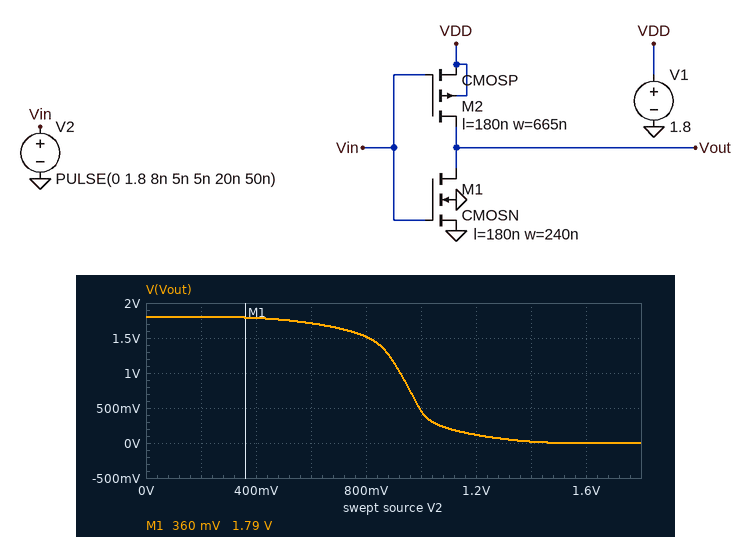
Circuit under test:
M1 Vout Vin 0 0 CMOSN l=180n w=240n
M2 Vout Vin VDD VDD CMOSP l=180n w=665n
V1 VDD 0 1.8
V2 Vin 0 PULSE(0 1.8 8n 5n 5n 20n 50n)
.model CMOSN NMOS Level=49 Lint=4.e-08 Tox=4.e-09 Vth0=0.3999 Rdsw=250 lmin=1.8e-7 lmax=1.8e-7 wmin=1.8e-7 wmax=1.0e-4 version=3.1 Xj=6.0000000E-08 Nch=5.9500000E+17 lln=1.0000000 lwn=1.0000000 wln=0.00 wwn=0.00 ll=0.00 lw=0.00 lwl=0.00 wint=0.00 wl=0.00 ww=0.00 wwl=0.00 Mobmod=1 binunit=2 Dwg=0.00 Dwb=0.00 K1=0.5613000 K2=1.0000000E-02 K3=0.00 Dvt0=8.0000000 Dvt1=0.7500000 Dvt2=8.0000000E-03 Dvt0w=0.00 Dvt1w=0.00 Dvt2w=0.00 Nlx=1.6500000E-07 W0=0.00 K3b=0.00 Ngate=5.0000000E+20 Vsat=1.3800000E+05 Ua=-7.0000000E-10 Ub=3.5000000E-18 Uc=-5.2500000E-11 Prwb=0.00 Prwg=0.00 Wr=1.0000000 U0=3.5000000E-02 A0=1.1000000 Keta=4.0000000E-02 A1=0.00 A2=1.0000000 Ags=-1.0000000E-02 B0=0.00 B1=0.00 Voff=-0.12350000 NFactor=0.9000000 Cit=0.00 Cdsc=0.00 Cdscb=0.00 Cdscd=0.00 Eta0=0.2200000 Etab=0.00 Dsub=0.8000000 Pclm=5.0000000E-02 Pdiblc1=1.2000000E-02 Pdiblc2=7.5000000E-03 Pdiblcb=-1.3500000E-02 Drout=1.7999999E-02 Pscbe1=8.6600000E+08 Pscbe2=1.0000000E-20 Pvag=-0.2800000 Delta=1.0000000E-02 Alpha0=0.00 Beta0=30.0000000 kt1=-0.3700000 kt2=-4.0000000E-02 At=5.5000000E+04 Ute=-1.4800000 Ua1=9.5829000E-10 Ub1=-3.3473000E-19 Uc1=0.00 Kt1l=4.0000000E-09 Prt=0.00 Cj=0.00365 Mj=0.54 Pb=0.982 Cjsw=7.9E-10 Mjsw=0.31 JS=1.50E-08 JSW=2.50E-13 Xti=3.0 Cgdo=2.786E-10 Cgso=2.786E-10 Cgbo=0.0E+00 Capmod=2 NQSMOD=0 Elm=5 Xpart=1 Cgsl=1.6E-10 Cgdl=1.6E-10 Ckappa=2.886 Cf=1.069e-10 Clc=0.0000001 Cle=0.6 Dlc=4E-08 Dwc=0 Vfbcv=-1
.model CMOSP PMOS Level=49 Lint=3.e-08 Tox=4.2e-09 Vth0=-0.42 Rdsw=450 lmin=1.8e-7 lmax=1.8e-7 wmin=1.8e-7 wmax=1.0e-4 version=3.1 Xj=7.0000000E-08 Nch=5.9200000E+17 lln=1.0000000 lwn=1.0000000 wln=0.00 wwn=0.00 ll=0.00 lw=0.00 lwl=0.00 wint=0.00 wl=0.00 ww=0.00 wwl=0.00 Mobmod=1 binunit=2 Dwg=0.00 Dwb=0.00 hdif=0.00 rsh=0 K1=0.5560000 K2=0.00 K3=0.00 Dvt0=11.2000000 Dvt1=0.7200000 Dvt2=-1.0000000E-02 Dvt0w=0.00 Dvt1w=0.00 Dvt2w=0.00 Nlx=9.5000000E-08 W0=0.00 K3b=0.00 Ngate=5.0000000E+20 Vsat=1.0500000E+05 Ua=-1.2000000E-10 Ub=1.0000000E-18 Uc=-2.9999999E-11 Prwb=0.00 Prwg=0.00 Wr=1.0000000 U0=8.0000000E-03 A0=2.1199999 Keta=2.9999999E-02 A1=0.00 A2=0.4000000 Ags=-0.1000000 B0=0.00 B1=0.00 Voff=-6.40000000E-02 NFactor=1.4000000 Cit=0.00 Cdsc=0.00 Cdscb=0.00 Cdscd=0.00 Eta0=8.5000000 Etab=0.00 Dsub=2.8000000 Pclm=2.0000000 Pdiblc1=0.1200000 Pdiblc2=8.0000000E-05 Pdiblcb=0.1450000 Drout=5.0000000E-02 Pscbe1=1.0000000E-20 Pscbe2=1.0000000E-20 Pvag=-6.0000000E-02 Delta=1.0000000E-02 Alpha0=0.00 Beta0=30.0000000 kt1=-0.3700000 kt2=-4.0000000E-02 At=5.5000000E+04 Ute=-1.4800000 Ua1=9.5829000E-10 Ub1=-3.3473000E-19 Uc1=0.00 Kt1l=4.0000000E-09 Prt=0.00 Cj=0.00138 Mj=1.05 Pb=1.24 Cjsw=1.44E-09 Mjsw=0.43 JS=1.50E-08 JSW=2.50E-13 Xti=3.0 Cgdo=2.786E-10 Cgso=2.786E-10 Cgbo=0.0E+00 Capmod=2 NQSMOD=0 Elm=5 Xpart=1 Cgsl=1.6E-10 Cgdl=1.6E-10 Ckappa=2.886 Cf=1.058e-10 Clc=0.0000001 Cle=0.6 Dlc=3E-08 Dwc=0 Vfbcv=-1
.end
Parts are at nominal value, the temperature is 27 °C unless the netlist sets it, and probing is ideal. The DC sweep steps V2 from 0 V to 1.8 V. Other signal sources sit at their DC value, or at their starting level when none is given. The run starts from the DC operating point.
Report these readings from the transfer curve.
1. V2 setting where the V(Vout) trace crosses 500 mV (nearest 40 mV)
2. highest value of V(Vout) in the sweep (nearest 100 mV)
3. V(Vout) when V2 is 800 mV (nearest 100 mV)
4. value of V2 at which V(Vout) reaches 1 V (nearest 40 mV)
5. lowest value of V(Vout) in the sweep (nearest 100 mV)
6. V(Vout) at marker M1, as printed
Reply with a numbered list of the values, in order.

1. 1.00 V
2. 1.8 V
3. 1.5 V
4. 920 mV
5. 0 V
6. 1.79 V
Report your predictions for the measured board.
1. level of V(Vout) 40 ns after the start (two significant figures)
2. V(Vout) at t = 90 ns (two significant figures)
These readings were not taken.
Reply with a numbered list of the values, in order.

1. 1.8 V
2. 1.8 V
